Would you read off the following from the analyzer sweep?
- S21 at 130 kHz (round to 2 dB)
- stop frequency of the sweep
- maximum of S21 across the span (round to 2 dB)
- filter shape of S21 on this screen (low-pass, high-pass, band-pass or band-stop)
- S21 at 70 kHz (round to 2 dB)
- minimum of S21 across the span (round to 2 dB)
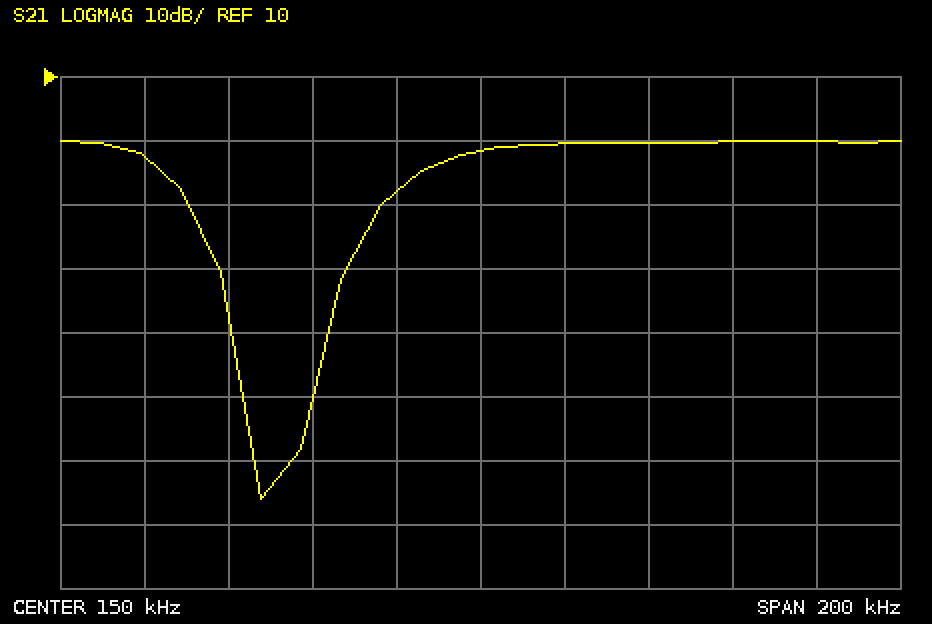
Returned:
-8 dB
250 kHz
0 dB
band-stop
-2 dB
-56 dB
